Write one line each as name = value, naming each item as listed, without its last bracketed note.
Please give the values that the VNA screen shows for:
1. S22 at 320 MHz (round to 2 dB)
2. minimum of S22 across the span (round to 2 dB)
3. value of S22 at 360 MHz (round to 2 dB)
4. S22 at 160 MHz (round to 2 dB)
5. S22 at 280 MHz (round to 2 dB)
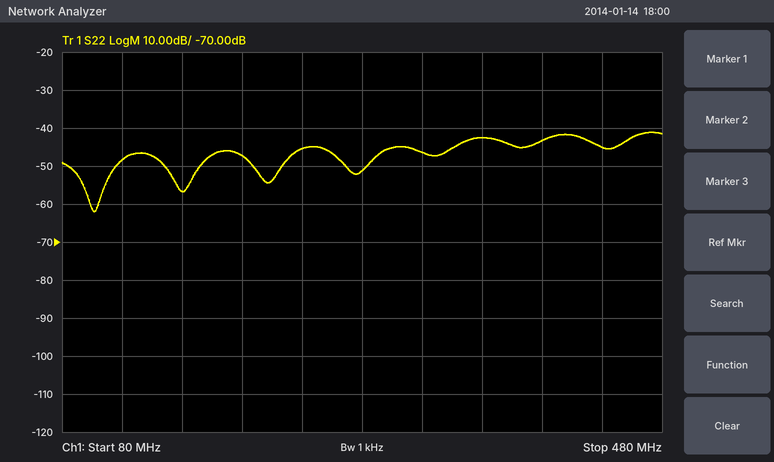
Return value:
S22 at 320 MHz = -46 dB
minimum of S22 across the span = -62 dB
value of S22 at 360 MHz = -42 dB
S22 at 160 MHz = -56 dB
S22 at 280 MHz = -52 dB
